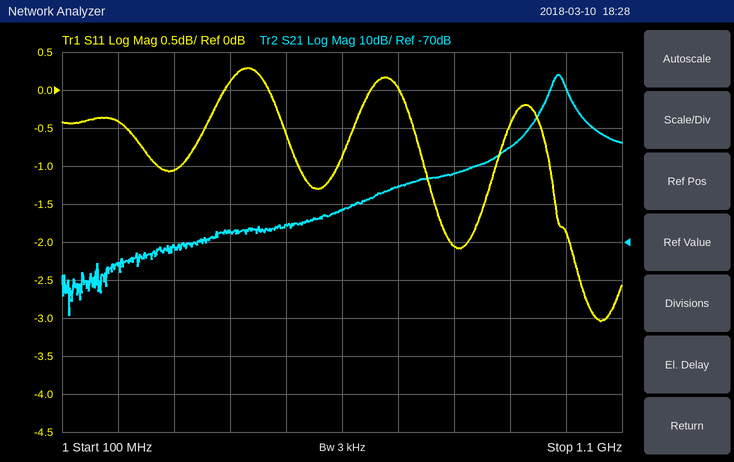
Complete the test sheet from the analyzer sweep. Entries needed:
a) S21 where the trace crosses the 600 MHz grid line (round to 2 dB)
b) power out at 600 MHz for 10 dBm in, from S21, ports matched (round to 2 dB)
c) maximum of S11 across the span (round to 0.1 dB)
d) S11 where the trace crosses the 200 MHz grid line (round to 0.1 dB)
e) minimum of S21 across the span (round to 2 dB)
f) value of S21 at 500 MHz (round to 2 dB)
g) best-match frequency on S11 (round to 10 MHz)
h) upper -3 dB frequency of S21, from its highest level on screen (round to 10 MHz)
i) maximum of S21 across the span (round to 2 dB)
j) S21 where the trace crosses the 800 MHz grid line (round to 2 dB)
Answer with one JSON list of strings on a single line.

["-62 dB", "-52 dBm", "0.3 dB", "-0.4 dB", "-90 dB", "-66 dB", "1.06 GHz", "1.00 GHz", "-26 dB", "-52 dB"]
